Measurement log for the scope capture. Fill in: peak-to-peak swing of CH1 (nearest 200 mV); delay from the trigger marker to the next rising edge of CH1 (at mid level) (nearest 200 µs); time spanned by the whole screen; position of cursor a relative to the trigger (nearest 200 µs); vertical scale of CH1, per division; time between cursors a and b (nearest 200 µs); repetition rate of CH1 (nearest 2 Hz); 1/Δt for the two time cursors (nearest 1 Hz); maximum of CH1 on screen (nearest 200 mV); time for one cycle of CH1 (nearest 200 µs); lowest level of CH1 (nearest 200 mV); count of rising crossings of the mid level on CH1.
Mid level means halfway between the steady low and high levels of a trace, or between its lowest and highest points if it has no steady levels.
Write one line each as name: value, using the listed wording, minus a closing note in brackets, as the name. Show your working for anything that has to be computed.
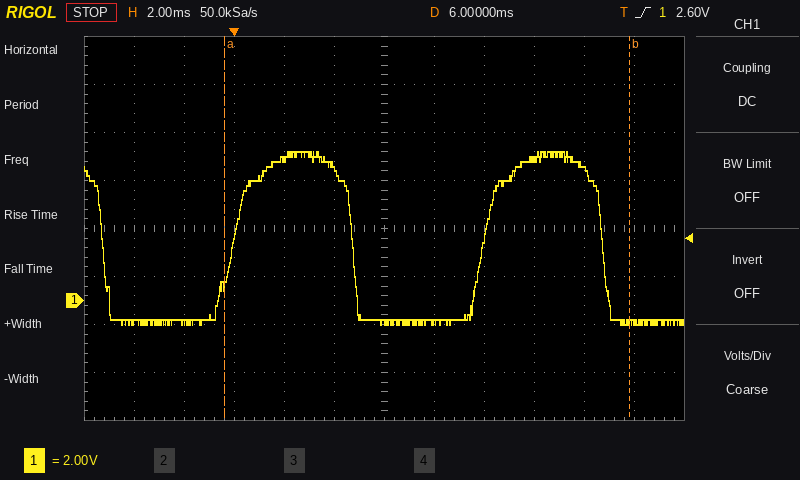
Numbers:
peak-to-peak swing of CH1: 6.2 V − (-1.0 V) = 7.2 V
delay from the trigger marker to the next rising edge of CH1 (at mid level): 10.0 ms
time spanned by the whole screen: 24 ms
position of cursor a relative to the trigger: -400 µs
vertical scale of CH1, per division: 2 V
time between cursors a and b: 16.2 ms
repetition rate of CH1: 1 / 10.0 ms ≈ 100 Hz
1/Δt for the two time cursors: 1 / 16.2 ms ≈ 62 Hz
maximum of CH1 on screen: 6.2 V
time for one cycle of CH1: 10.0 ms
lowest level of CH1: -1.0 V
count of rising crossings of the mid level on CH1: 2
